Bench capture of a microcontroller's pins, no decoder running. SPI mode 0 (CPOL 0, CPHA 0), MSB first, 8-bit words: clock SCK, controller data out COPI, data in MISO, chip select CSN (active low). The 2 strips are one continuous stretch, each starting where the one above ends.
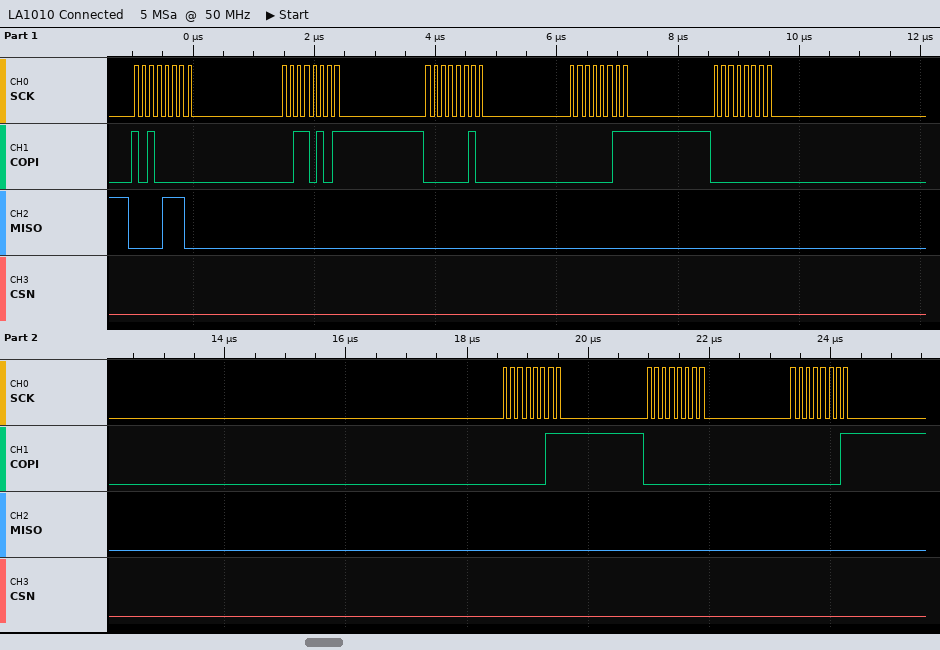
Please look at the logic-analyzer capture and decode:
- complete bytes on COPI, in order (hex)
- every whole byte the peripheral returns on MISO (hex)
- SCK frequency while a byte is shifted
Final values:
A0 35 02 03 00 03 00 01
0E 00 00 00 00 00 00 00
8 MHz
